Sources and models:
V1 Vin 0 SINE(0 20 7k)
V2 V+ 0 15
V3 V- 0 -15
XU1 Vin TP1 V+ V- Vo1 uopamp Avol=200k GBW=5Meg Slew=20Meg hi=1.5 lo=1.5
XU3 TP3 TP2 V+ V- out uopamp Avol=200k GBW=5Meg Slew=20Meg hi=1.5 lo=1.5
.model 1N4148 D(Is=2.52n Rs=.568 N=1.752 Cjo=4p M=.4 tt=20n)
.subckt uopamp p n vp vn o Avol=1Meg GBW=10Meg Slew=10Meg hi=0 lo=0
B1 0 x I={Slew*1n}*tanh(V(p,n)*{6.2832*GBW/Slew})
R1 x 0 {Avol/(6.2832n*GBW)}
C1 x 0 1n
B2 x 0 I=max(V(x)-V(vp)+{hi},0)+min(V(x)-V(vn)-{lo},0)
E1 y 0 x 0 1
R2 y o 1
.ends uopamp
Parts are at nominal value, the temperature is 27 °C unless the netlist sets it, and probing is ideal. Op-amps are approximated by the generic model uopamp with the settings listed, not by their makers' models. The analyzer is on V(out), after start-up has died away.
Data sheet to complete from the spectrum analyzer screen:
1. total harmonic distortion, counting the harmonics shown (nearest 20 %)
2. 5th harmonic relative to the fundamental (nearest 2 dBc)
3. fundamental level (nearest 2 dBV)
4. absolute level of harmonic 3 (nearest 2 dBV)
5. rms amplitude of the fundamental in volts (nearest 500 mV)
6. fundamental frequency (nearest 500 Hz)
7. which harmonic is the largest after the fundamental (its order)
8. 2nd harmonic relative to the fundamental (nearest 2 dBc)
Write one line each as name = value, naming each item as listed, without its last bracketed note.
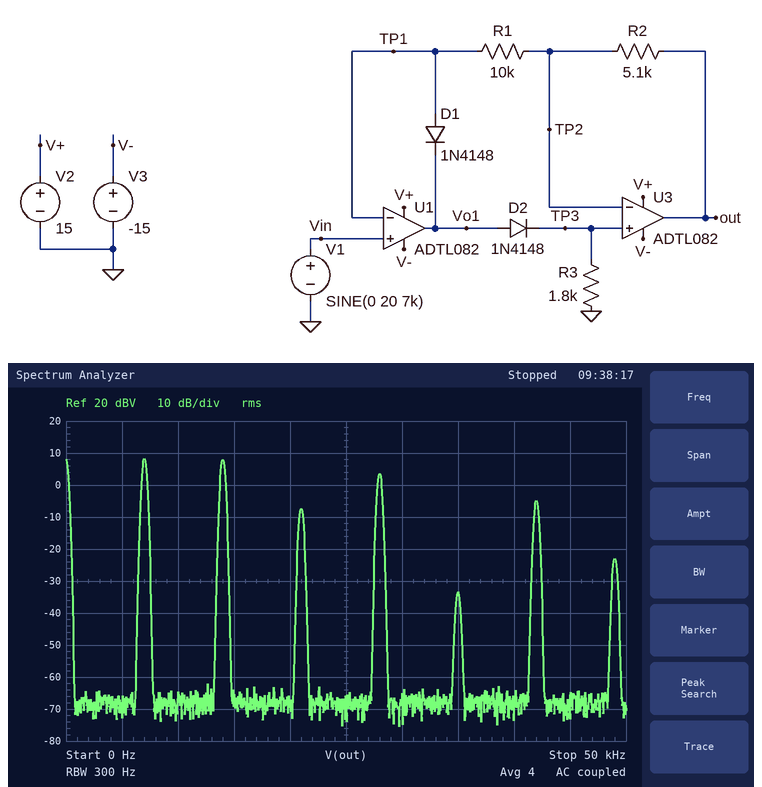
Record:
total harmonic distortion, counting the harmonics shown = 120 %
5th harmonic relative to the fundamental = -42 dBc
fundamental level = 8 dBV
absolute level of harmonic 3 = -8 dBV
rms amplitude of the fundamental in volts = 2.5 V
fundamental frequency = 7.0 kHz
which harmonic is the largest after the fundamental = 2
2nd harmonic relative to the fundamental = 0 dBc
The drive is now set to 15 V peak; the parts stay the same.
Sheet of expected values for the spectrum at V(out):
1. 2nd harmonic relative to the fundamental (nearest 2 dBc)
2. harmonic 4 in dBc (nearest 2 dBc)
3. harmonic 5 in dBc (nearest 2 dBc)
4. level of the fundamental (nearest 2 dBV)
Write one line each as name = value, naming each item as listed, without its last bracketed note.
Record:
2nd harmonic relative to the fundamental = 2 dBc
harmonic 4 in dBc = -8 dBc
harmonic 5 in dBc = -30 dBc
level of the fundamental = 8 dBV
